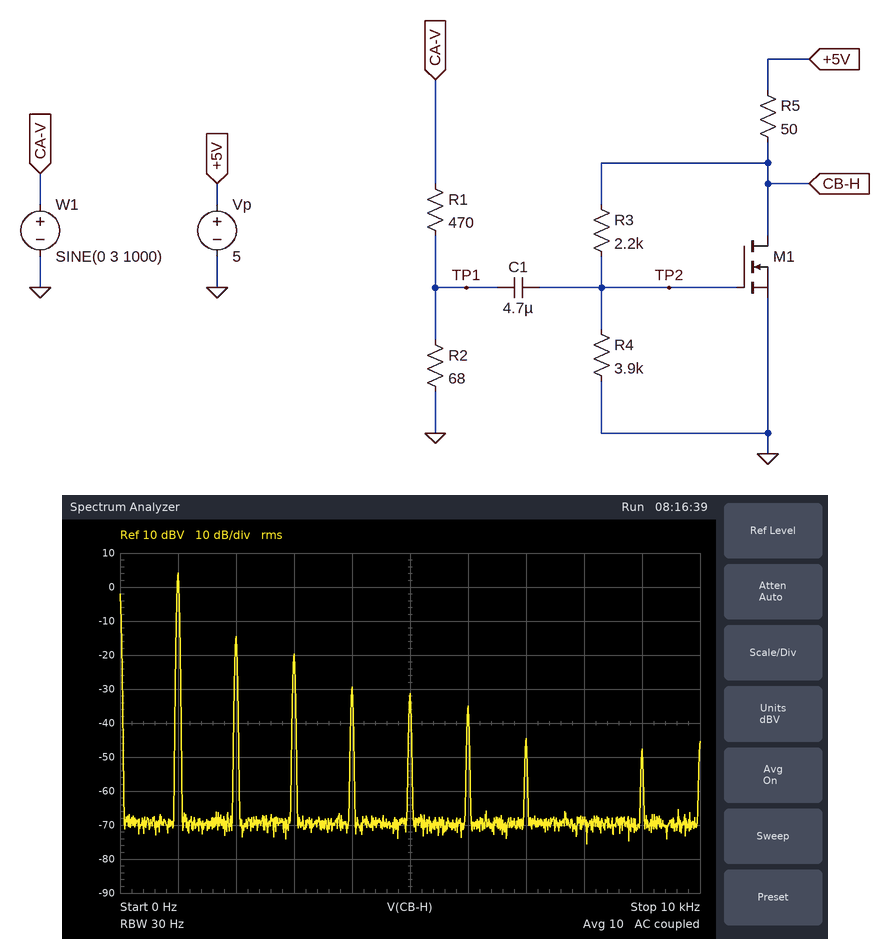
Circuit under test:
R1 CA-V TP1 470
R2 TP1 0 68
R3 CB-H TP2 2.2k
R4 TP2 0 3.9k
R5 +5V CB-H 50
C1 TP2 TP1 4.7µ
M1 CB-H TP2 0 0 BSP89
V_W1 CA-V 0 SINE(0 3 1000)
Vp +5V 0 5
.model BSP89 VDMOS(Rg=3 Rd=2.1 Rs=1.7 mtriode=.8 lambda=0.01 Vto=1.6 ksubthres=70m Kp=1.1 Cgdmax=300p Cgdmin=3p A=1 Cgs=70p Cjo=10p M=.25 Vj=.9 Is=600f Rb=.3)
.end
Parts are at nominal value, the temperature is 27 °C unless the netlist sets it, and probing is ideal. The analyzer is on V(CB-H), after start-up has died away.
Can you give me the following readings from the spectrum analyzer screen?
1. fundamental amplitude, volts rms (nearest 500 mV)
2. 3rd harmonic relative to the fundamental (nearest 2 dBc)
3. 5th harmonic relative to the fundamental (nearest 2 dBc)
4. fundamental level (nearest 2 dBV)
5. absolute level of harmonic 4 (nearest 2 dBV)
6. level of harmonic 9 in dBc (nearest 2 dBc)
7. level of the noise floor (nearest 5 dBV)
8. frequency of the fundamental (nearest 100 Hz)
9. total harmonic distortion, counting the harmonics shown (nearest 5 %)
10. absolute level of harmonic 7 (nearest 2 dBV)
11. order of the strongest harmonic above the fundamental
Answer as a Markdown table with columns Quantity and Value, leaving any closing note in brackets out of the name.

| Quantity | Value |
|---|---|
| fundamental amplitude, volts rms | 1.5 V |
| 3rd harmonic relative to the fundamental | -24 dBc |
| 5th harmonic relative to the fundamental | -36 dBc |
| fundamental level | 4 dBV |
| absolute level of harmonic 4 | -30 dBV |
| level of harmonic 9 in dBc | -52 dBc |
| level of the noise floor | -70 dBV |
| frequency of the fundamental | 1.0 kHz |
| total harmonic distortion, counting the harmonics shown | 15 % |
| absolute level of harmonic 7 | -44 dBV |
| order of the strongest harmonic above the fundamental | 2 |
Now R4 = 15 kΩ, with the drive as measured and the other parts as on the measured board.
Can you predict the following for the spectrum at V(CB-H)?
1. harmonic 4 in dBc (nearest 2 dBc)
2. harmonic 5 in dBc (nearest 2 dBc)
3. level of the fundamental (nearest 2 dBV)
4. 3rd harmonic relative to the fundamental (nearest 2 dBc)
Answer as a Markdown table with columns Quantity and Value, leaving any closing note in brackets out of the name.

| Quantity | Value |
|---|---|
| harmonic 4 in dBc | -40 dBc |
| harmonic 5 in dBc | -34 dBc |
| level of the fundamental | 4 dBV |
| 3rd harmonic relative to the fundamental | -18 dBc |
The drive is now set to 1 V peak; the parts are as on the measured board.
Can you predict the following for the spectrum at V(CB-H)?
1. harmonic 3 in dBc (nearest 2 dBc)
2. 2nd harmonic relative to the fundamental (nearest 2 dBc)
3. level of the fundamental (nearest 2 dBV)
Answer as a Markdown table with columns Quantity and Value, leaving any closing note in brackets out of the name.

| Quantity | Value |
|---|---|
| harmonic 3 in dBc | -52 dBc |
| 2nd harmonic relative to the fundamental | -30 dBc |
| level of the fundamental | -4 dBV |
